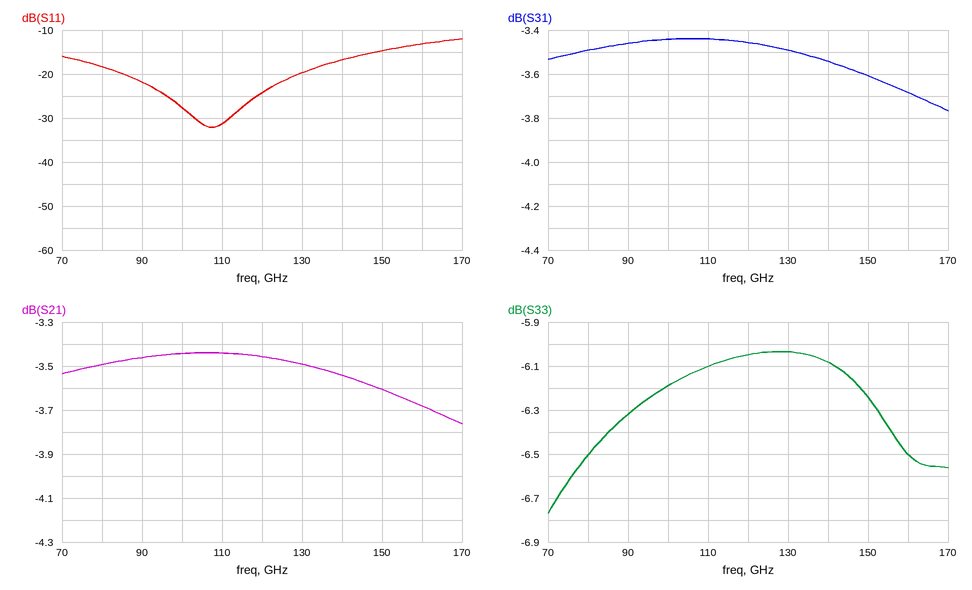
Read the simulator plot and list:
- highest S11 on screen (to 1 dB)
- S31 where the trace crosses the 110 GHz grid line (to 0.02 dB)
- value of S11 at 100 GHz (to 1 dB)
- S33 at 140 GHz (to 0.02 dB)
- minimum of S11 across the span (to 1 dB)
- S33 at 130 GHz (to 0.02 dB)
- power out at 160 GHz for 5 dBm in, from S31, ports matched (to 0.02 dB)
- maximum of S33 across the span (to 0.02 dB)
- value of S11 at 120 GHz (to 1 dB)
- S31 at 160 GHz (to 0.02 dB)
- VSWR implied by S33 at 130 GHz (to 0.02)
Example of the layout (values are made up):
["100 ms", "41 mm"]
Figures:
["-12 dB", "-3.44 dB", "-28 dB", "-6.08 dB", "-32 dB", "-6.04 dB", "1.32 dBm", "-6.04 dB", "-24 dB", "-3.68 dB", "3.00"]
